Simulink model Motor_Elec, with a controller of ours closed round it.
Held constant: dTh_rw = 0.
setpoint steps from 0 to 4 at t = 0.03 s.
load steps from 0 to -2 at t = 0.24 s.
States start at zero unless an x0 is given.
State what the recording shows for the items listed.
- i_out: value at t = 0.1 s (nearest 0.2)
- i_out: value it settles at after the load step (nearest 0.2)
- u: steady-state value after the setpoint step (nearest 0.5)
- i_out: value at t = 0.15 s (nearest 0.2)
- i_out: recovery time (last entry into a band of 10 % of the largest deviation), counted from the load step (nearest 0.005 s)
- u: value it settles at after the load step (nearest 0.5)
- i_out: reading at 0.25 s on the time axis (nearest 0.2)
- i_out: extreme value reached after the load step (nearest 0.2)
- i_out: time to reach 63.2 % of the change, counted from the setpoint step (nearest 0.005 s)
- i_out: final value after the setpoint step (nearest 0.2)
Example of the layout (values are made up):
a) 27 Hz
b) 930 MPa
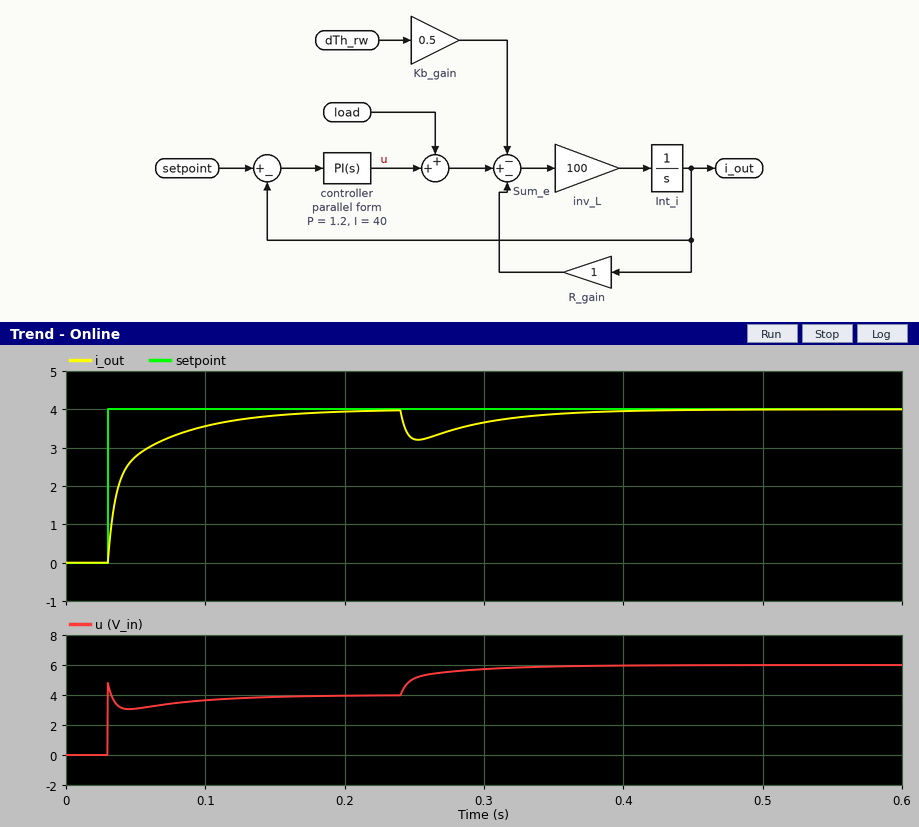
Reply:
a) 3.6
b) 4.0
c) 4.0
d) 3.8
e) 0.135 s
f) 6.0
g) 3.2
h) 3.2
i) 0.015 s
j) 4.0
